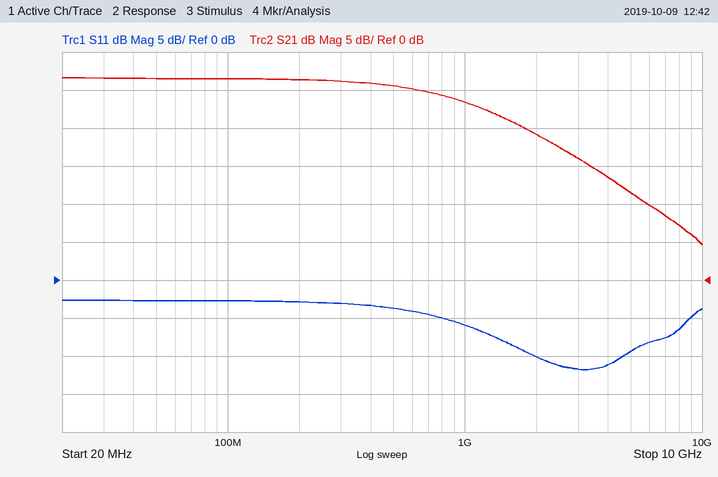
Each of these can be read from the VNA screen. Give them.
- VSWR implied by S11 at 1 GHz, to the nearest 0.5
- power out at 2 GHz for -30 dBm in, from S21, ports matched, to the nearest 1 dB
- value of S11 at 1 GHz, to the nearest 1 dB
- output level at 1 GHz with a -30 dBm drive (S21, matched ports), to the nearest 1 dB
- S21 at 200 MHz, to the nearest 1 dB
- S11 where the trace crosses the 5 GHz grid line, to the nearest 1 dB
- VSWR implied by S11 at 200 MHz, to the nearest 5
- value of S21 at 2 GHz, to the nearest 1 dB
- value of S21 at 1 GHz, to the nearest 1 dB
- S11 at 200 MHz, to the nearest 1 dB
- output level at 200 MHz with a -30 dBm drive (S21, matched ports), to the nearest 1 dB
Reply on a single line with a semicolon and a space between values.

3.0; -11 dBm; -6 dB; -7 dBm; 26 dB; -9 dB; 5; 19 dB; 23 dB; -3 dB; -4 dBm
